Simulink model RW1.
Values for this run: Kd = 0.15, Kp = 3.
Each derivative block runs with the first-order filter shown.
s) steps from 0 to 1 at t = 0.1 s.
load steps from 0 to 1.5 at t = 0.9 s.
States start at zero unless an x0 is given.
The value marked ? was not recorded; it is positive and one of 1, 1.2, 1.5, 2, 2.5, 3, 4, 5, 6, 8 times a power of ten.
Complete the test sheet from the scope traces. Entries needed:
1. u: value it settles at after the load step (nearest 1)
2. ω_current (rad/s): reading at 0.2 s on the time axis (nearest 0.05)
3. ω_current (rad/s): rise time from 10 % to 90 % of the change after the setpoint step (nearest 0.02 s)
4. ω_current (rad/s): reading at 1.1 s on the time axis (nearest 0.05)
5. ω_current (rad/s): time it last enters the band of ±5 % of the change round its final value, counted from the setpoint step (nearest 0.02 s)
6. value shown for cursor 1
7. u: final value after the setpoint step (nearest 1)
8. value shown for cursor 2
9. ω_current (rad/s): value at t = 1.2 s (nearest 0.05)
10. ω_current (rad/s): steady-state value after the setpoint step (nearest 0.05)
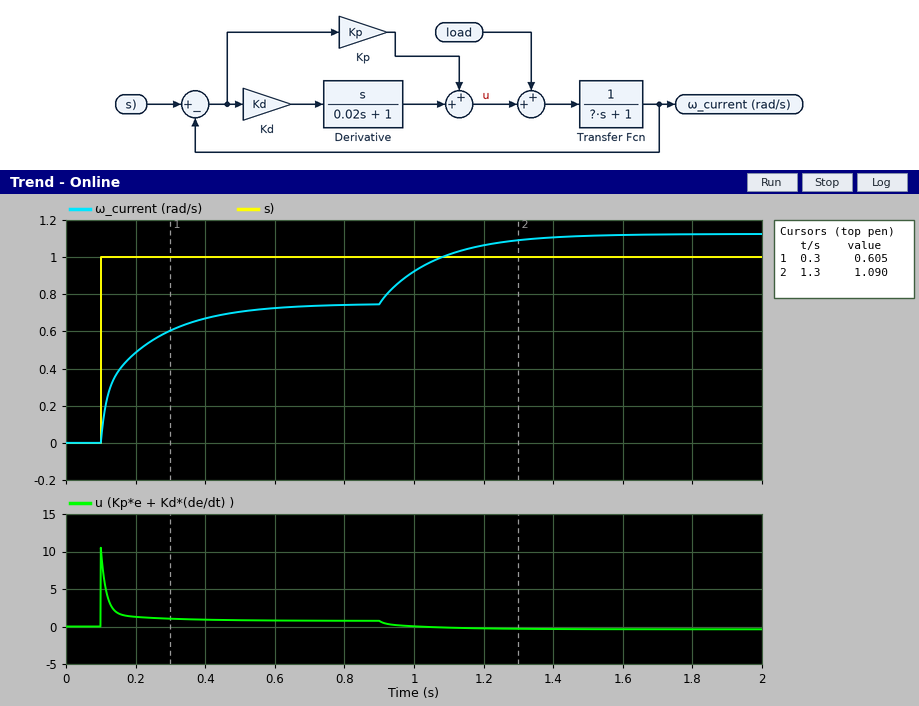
0
0.50
0.30 s
1.00
0.42 s
0.605
1
1.090
1.05
0.75
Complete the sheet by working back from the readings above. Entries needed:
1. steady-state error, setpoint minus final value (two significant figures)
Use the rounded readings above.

0.25
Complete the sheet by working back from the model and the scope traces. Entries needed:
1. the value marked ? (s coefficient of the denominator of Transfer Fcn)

0.5
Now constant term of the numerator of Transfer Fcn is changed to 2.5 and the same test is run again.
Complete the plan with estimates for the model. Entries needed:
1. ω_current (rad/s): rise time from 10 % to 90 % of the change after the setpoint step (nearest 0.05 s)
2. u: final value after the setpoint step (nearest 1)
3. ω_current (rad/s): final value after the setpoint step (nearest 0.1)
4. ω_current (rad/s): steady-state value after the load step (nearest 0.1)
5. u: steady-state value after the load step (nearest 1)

0.15 s
0
0.9
1.3
-1
